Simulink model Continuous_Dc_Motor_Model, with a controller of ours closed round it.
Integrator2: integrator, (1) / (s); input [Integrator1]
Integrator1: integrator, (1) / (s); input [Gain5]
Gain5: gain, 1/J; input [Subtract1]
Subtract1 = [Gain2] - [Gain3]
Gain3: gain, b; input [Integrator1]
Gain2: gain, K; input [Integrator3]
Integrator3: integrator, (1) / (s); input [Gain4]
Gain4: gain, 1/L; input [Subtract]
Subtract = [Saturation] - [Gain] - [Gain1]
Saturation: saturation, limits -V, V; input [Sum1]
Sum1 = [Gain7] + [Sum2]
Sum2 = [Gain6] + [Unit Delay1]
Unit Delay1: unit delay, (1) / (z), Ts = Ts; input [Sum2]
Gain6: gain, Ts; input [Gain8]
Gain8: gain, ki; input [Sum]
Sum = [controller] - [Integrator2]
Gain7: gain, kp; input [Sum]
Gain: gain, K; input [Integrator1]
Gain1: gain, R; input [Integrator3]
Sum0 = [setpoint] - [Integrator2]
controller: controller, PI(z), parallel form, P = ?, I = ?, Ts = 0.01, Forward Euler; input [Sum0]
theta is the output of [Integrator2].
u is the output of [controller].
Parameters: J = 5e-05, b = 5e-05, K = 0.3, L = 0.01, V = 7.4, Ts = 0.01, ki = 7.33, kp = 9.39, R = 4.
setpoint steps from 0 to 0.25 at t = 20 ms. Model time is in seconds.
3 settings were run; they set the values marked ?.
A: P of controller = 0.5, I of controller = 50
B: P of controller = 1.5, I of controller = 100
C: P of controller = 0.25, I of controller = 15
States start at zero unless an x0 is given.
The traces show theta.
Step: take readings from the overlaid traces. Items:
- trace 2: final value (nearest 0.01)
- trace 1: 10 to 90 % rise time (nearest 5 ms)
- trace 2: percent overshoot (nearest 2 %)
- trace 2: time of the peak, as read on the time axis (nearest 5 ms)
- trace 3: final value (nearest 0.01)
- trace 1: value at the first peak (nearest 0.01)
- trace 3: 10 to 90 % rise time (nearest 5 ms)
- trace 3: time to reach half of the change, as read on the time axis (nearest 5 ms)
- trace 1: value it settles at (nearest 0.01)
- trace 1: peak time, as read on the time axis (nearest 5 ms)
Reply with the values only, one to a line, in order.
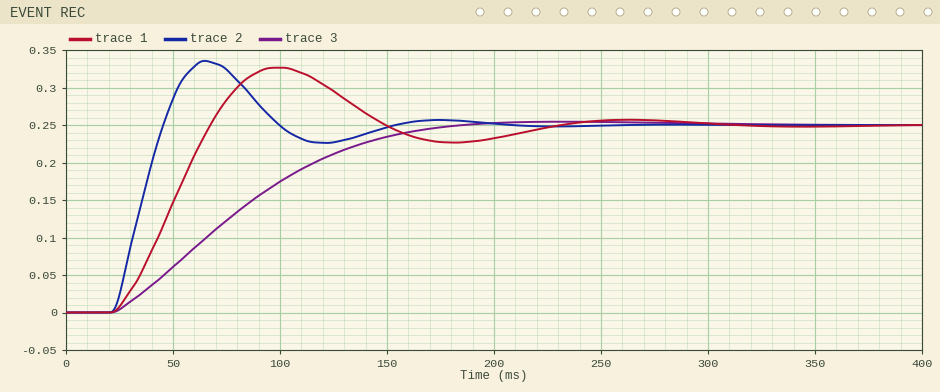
0.25
35 ms
34 %
65 ms
0.25
0.33
105 ms
75 ms
0.25
100 ms
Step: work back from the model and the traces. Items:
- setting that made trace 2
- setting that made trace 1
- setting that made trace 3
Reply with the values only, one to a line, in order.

B
A
C
